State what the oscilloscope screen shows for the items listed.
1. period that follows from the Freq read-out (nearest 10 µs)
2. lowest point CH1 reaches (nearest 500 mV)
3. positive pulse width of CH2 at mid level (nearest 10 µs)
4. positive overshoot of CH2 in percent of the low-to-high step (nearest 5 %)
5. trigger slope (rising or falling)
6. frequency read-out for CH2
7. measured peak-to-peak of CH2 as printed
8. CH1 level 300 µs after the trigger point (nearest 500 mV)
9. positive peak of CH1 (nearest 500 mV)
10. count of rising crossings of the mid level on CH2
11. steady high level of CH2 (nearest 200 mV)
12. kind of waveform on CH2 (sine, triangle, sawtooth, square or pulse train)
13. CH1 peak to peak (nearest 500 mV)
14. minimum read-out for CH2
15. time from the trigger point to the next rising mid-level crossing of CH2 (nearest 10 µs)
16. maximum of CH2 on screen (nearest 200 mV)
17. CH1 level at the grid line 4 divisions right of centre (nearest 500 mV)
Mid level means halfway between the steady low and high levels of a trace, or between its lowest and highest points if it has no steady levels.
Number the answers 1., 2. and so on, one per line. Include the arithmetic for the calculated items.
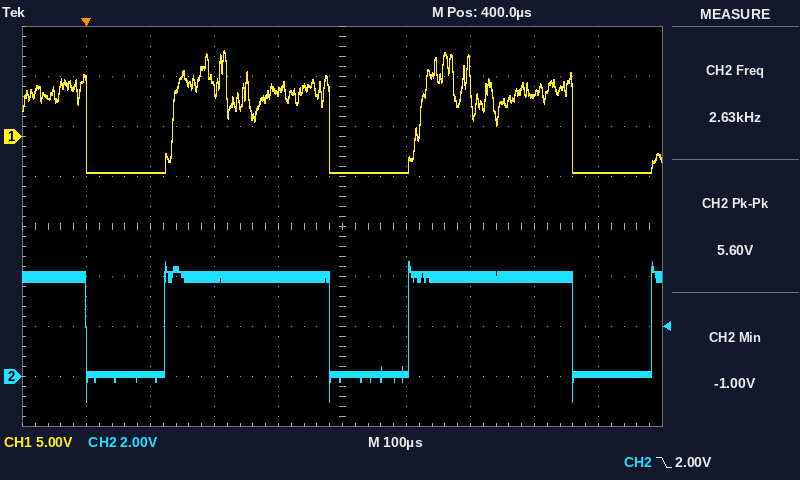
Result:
1. 1 / 2.63 kHz ≈ 380 µs
2. -3.5 V
3. 260 µs
4. 15 %
5. falling
6. 2.63 kHz
7. 5.60 V
8. 4.5 V
9. 8.5 V
10. 3
11. 4.0 V
12. pulse train
13. 8.5 V − (-3.5 V) = 12.0 V
14. -1.00 V
15. 120 µs
16. 4.6 V
17. -3.5 V
